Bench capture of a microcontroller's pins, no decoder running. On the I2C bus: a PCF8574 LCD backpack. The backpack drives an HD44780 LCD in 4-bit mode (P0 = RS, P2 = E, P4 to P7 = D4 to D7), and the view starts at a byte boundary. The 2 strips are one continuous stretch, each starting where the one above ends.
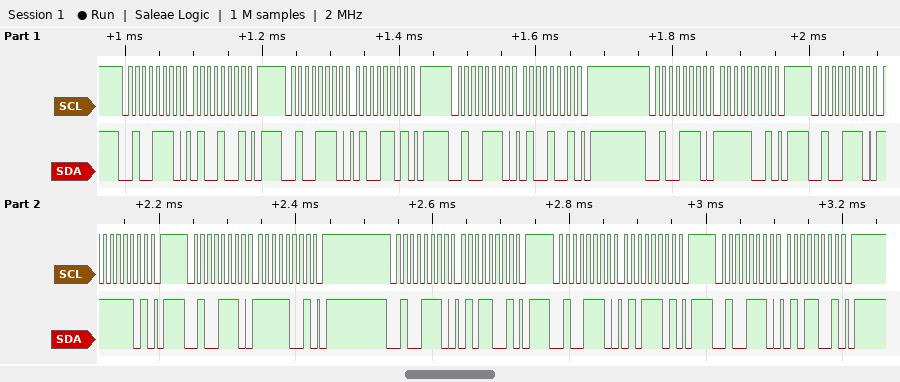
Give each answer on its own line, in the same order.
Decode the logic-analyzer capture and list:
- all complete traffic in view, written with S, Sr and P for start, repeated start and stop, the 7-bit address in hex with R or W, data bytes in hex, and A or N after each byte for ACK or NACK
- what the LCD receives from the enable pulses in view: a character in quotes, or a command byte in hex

S 27W A 49 A P S 27W A 4D A P S 27W A 49 A P S 27W A F9 A P S 27W A FD A P S 27W A F9 A P S 27W A 59 A P S 27W A 5D A P S 27W A 59 A P
'O'
